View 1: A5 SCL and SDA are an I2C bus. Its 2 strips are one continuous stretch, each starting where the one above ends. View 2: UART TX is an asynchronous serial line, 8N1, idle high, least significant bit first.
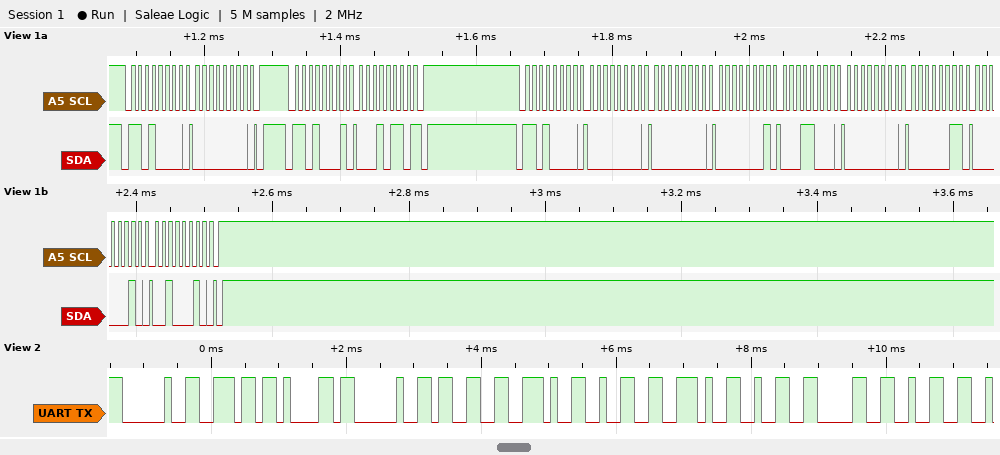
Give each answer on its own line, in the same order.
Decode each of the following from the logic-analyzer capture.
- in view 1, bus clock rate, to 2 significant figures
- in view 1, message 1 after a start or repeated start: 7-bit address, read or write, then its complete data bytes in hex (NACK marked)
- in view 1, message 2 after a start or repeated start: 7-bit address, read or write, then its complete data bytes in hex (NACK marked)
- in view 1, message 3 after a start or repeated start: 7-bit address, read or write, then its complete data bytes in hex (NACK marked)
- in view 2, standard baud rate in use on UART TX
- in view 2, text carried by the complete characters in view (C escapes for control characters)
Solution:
100 kHz
0x68 write: 00
0x68 read: 16 NACK
0x68 write: 00 00 01 18 00 03 02 22
9600 baud
" na 3.2.202"
